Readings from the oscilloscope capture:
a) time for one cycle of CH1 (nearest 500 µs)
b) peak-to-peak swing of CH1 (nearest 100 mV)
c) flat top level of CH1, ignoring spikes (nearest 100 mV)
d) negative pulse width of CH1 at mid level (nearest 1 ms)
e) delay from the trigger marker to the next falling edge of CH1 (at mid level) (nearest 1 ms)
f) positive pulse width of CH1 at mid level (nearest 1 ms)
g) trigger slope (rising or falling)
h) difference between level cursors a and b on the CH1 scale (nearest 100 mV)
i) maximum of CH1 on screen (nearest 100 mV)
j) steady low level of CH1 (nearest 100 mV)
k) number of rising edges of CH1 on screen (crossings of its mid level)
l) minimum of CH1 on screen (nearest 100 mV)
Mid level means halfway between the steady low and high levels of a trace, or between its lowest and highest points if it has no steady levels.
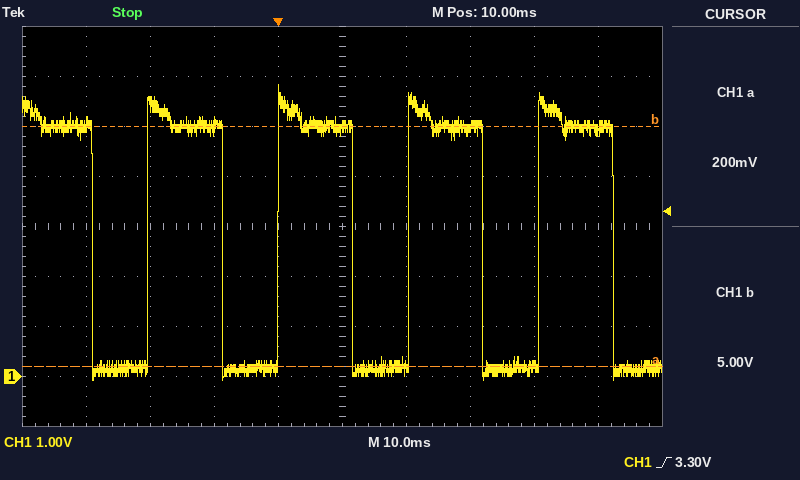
20.5 ms
5.9 V
5.0 V
9 ms
12 ms
12 ms
rising
4.8 V
5.8 V
200 mV
4
-100 mV
